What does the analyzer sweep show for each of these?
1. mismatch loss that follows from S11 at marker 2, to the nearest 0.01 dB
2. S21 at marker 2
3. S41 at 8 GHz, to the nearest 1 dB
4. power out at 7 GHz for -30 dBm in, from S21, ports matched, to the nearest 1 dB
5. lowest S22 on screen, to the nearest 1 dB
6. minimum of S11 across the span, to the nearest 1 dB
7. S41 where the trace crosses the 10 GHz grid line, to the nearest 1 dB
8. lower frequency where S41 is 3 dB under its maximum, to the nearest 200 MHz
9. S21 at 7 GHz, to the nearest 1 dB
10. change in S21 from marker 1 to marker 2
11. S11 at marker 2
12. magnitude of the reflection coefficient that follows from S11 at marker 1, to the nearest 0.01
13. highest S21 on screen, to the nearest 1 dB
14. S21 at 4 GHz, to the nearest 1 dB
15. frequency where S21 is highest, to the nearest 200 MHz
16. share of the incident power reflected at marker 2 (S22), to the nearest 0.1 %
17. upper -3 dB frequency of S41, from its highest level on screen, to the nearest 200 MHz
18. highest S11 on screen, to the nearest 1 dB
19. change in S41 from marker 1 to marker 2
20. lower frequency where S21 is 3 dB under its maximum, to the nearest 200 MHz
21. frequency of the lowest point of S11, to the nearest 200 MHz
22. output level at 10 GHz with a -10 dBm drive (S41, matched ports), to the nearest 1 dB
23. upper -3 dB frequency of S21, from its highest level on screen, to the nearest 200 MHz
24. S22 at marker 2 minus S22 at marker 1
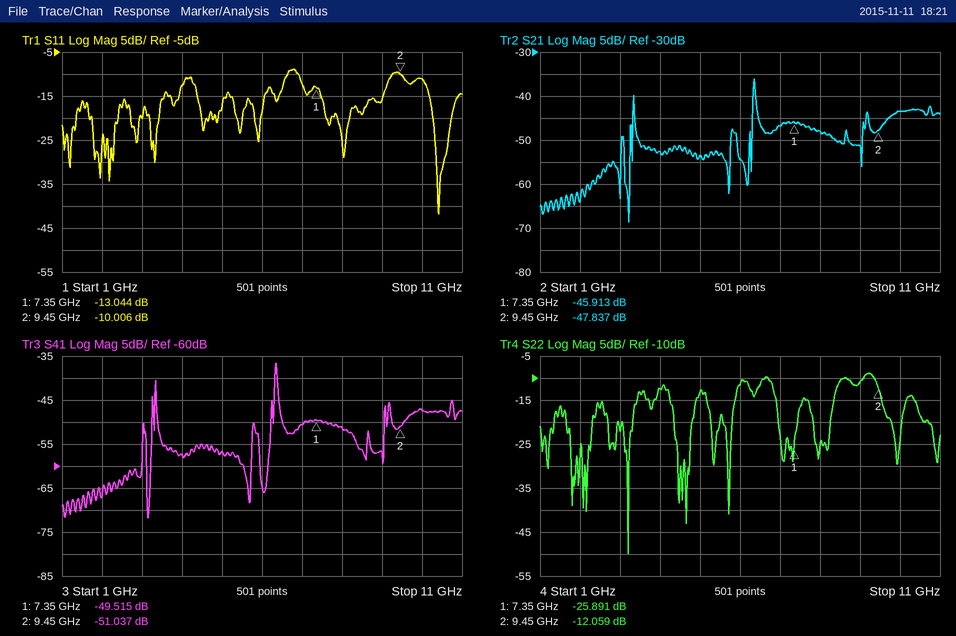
0.46 dB
-47.837 dB
-51 dB
-77 dBm
-50 dB
-42 dB
-47 dB
6.4 GHz
-47 dB
-1.924 dB
-10.006 dB
0.22
-36 dB
-53 dB
6.4 GHz
6.2 %
6.4 GHz
-9 dB
-1.522 dB
6.4 GHz
10.4 GHz
-57 dBm
6.4 GHz
13.832 dB
